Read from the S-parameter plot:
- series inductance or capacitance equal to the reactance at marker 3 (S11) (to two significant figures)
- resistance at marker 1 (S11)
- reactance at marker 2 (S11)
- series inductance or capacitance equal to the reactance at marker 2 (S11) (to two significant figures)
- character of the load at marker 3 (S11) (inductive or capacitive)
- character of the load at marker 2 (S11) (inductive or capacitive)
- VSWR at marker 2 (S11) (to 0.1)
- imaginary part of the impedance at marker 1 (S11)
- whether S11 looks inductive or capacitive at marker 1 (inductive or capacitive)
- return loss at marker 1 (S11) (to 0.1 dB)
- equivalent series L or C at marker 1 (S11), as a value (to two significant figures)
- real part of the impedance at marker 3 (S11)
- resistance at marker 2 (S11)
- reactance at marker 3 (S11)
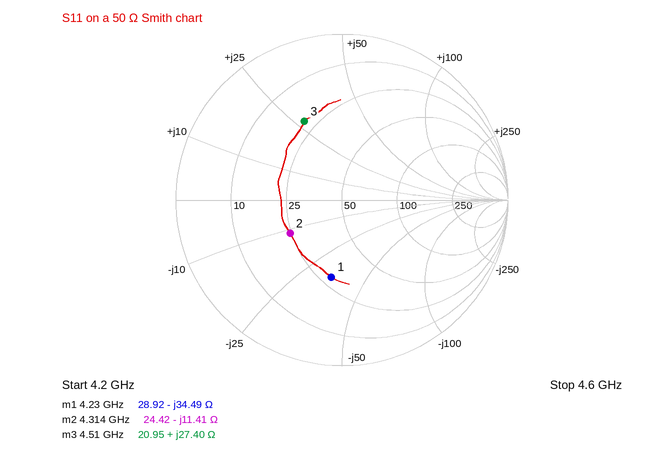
970 pH
28.92 Ω
-11.41 Ω
3.2 pF
inductive
capacitive
2.2
-34.49 Ω
capacitive
6.6 dB
1.1 pF
20.95 Ω
24.42 Ω
+27.40 Ω
